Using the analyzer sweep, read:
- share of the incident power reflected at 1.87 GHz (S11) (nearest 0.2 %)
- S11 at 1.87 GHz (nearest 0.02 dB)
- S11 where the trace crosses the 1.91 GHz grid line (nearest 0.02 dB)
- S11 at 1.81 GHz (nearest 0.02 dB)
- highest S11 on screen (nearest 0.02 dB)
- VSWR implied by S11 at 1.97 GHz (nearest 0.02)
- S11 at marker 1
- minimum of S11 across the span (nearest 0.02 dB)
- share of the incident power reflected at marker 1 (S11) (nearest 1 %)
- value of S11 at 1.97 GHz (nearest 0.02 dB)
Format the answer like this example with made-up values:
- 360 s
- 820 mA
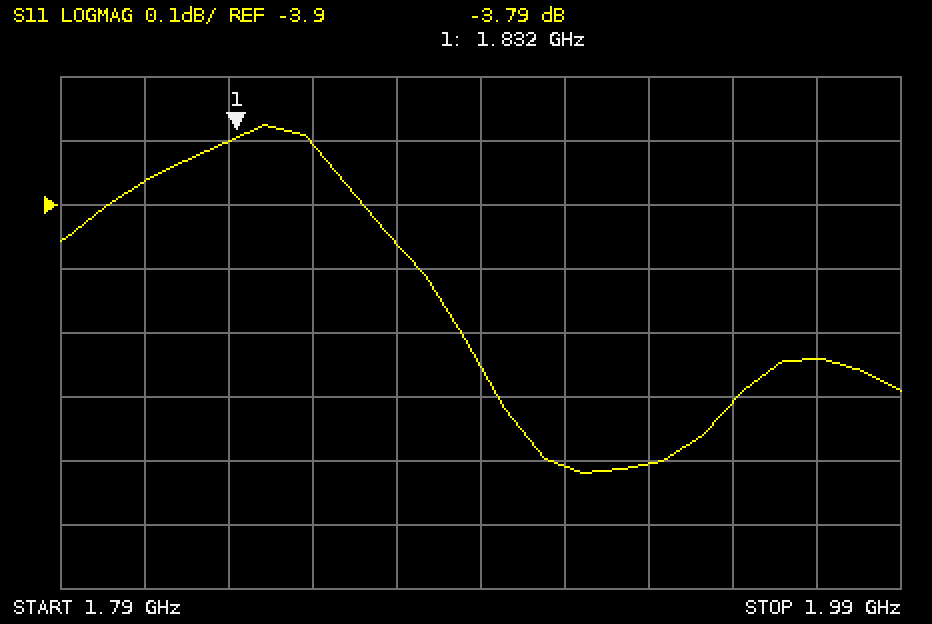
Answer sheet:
- 40.2 %
- -3.96 dB
- -4.30 dB
- -3.86 dB
- -3.78 dB
- 4.28
- -3.79 dB
- -4.32 dB
- 42 %
- -4.14 dB
